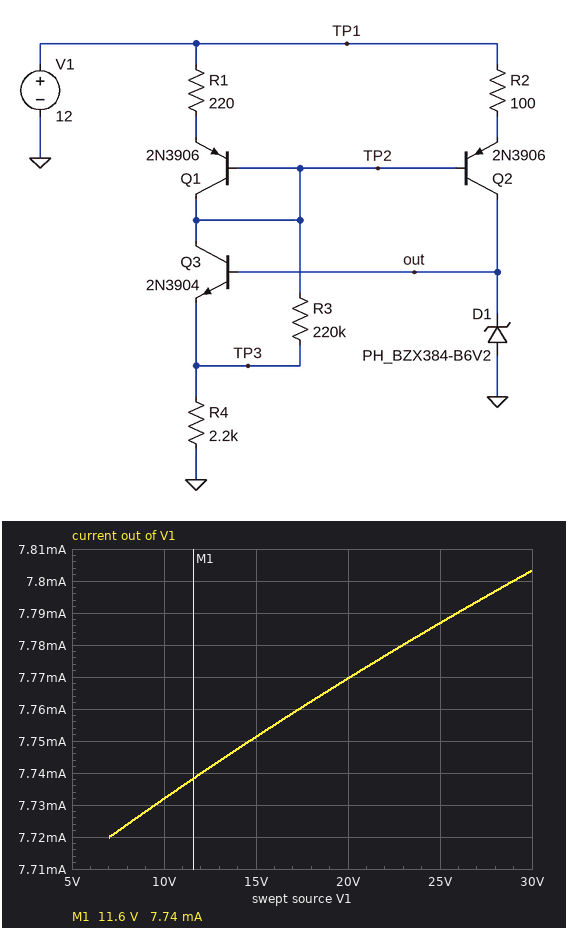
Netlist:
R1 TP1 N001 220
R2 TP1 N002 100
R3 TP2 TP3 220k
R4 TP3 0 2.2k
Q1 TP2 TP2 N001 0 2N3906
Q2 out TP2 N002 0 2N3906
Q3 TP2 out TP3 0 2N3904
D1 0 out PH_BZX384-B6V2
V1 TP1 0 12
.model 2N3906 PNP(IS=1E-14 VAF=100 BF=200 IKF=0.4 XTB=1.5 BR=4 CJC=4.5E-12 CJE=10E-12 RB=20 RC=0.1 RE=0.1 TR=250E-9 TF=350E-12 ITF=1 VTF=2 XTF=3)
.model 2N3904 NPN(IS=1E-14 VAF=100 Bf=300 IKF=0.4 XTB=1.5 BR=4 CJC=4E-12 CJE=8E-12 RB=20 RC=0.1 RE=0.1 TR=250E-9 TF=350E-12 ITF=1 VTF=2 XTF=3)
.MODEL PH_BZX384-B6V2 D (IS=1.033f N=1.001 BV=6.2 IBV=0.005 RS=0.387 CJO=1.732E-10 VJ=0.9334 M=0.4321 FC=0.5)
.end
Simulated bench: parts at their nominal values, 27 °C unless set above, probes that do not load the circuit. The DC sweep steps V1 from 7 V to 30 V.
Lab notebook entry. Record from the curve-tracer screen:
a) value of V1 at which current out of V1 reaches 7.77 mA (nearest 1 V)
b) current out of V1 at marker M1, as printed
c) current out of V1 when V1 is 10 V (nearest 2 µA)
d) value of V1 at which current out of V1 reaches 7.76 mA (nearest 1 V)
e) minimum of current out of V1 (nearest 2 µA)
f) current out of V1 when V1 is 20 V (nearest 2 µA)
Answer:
20 V
7.74 mA
7.732 mA
17 V
7.720 mA
7.770 mA
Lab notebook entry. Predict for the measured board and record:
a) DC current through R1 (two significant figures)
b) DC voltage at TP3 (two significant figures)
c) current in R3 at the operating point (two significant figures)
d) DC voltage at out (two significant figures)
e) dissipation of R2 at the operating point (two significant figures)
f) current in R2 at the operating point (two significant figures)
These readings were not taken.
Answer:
2.5 mA
5.5 V
24 µA
6.2 V
2.8 mW
5.3 mA
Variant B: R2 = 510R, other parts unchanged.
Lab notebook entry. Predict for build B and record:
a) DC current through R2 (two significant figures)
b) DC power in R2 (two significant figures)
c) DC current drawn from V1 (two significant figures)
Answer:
1.1 mA
630 µW
3.6 mA
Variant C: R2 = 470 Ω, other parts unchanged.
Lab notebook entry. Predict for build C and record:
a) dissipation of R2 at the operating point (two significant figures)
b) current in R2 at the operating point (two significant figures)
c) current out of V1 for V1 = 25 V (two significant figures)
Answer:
680 µW
1.2 mA
3.7 mA
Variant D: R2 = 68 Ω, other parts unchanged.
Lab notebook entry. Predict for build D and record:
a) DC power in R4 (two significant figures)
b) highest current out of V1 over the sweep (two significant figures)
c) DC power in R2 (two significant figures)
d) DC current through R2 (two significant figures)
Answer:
14 mW
10 mA
3.9 mW
7.6 mA
